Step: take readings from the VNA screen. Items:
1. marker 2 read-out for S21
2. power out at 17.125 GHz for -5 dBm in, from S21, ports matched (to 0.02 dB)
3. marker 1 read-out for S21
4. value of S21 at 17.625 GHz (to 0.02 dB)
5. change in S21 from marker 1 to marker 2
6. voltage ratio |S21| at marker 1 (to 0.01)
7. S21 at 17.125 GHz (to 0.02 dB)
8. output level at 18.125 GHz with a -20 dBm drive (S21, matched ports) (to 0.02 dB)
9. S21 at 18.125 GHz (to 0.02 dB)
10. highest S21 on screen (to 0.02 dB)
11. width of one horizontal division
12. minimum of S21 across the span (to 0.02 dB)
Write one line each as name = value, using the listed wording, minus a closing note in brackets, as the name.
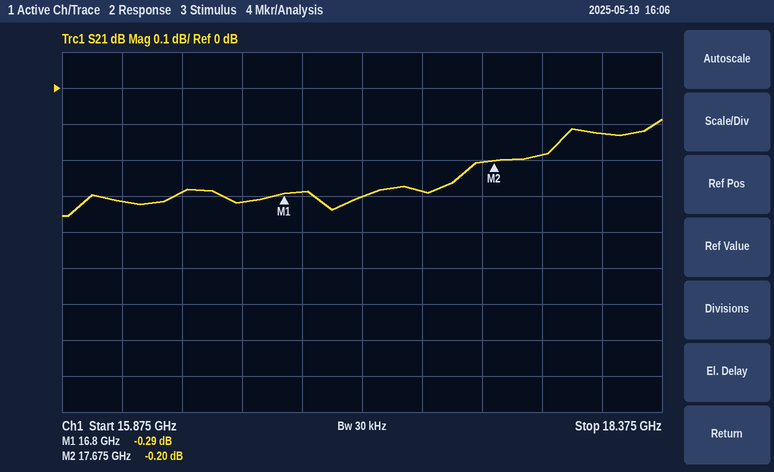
marker 2 read-out for S21 = -0.20 dB
power out at 17.125 GHz for -5 dBm in, from S21, ports matched = -5.30 dBm
marker 1 read-out for S21 = -0.29 dB
value of S21 at 17.625 GHz = -0.20 dB
change in S21 from marker 1 to marker 2 = 0.09 dB
voltage ratio |S21| at marker 1 = 0.97
S21 at 17.125 GHz = -0.30 dB
output level at 18.125 GHz with a -20 dBm drive (S21, matched ports) = -20.12 dBm
S21 at 18.125 GHz = -0.12 dB
highest S21 on screen = -0.08 dB
width of one horizontal division = 250 MHz
minimum of S21 across the span = -0.36 dB
